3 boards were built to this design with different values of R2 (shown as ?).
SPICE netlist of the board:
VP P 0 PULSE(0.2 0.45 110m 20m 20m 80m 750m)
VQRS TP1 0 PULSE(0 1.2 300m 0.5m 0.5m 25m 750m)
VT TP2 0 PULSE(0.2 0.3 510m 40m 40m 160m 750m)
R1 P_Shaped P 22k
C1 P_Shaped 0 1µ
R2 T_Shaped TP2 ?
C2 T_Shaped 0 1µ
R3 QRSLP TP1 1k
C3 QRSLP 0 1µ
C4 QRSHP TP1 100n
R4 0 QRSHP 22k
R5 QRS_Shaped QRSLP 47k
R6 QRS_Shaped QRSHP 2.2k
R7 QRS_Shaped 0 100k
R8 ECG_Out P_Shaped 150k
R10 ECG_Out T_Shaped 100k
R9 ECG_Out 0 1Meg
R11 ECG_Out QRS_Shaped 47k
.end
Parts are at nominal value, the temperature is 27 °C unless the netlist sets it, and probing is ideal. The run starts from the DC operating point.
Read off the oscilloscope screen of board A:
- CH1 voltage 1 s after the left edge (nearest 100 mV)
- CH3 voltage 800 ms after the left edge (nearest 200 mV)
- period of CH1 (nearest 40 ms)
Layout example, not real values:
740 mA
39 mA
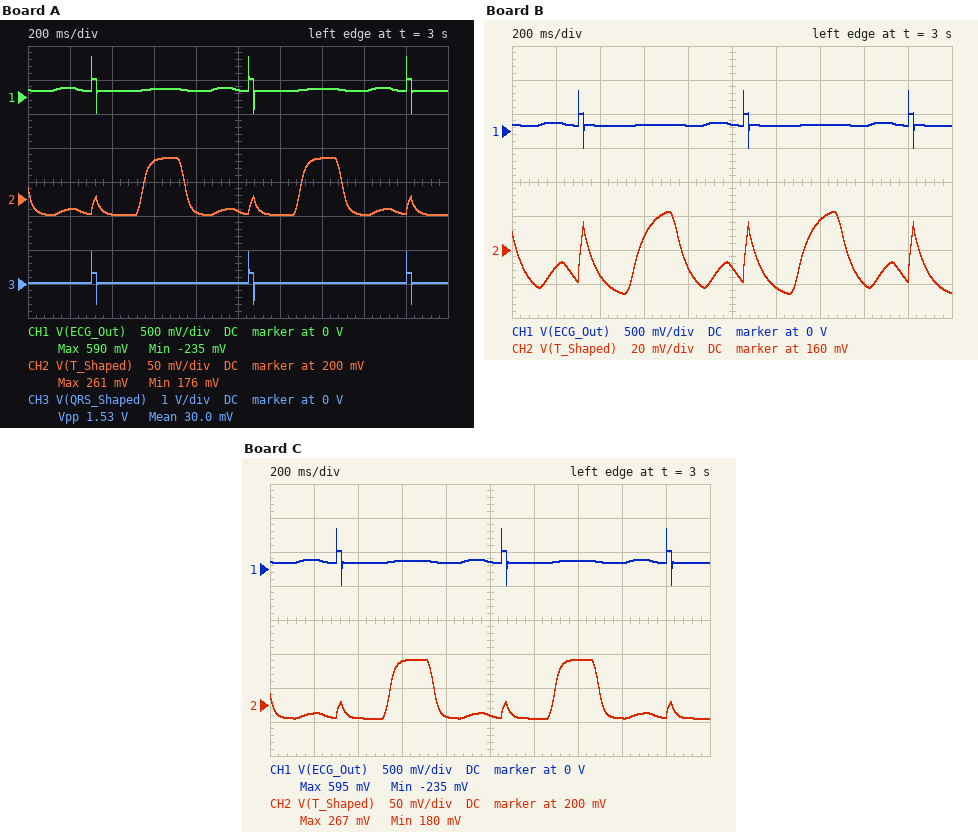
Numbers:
100 mV
0 V
760 ms
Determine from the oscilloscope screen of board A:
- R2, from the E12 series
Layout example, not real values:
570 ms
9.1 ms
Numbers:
27 kΩ
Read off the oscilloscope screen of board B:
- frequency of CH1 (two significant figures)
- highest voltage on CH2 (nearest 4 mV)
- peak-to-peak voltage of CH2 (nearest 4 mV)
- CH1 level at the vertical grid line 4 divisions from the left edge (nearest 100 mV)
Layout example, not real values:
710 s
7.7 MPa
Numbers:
1.3 Hz
184 mV
48 mV
100 mV
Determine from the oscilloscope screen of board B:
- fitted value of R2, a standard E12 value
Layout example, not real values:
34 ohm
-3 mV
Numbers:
120 kΩ
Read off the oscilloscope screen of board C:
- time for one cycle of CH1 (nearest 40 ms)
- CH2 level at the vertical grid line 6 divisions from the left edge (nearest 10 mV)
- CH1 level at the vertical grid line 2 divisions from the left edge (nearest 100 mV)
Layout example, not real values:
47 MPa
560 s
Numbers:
760 ms
180 mV
100 mV
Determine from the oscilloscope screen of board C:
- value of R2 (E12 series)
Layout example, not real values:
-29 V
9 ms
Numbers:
22 kΩ
